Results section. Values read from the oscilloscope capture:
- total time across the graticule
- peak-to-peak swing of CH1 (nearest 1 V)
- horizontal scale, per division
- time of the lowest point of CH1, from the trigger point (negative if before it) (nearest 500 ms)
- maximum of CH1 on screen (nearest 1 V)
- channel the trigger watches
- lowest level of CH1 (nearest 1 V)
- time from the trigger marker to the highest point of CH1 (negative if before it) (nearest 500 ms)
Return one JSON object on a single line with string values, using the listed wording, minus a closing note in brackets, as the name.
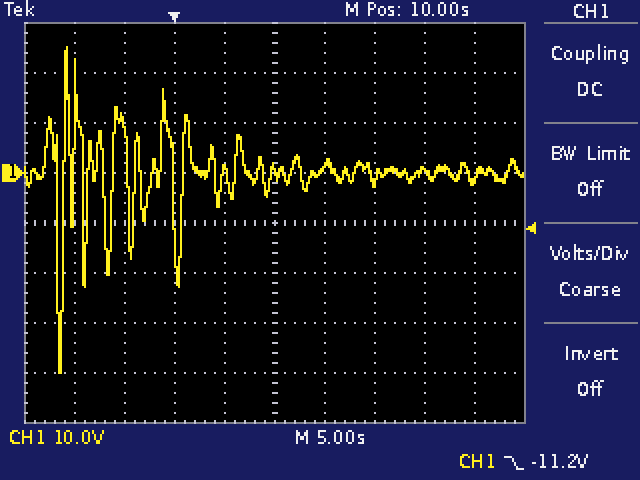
{"total time across the graticule": "50 s", "peak-to-peak swing of CH1": "65 V", "horizontal scale, per division": "5 s", "time of the lowest point of CH1, from the trigger point (negative if before it)": "-11.5 s", "maximum of CH1 on screen": "25 V", "channel the trigger watches": "CH1", "lowest level of CH1": "-40 V", "time from the trigger marker to the highest point of CH1 (negative if before it)": "-11.0 s"}
